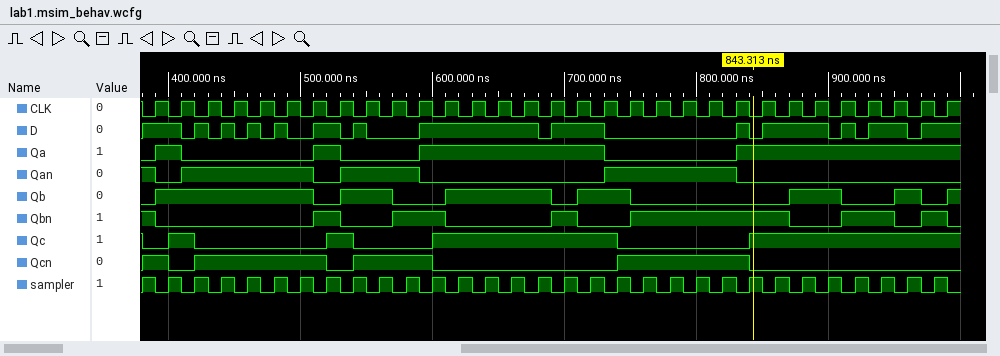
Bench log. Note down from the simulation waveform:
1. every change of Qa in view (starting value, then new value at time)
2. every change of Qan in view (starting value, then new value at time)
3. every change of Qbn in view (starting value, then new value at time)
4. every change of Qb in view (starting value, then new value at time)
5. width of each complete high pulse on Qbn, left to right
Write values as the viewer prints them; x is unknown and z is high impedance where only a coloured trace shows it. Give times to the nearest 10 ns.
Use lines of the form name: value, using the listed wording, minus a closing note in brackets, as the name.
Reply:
every change of Qa in view: 0, 1 at 390 ns, 0 at 410 ns, 1 at 510 ns, 0 at 530 ns, 1 at 590 ns, 0 at 730 ns, 1 at 830 ns
every change of Qan in view: 1, 0 at 390 ns, 1 at 410 ns, 0 at 510 ns, 1 at 530 ns, 0 at 590 ns, 1 at 730 ns, 0 at 830 ns
every change of Qbn in view: 1, 0 at 390 ns, 1 at 510 ns, 0 at 530 ns, 1 at 570 ns, 0 at 610 ns, 1 at 690 ns, 0 at 710 ns, 1 at 750 ns, 0 at 870 ns, 1 at 910 ns, 0 at 950 ns, 1 at 970 ns, 0 at 990 ns
every change of Qb in view: 0, 1 at 390 ns, 0 at 510 ns, 1 at 530 ns, 0 at 570 ns, 1 at 610 ns, 0 at 690 ns, 1 at 710 ns, 0 at 750 ns, 1 at 870 ns, 0 at 910 ns, 1 at 950 ns, 0 at 970 ns, 1 at 990 ns
width of each complete high pulse on Qbn, left to right: 20 ns, 40 ns, 20 ns, 120 ns, 40 ns, 20 ns
